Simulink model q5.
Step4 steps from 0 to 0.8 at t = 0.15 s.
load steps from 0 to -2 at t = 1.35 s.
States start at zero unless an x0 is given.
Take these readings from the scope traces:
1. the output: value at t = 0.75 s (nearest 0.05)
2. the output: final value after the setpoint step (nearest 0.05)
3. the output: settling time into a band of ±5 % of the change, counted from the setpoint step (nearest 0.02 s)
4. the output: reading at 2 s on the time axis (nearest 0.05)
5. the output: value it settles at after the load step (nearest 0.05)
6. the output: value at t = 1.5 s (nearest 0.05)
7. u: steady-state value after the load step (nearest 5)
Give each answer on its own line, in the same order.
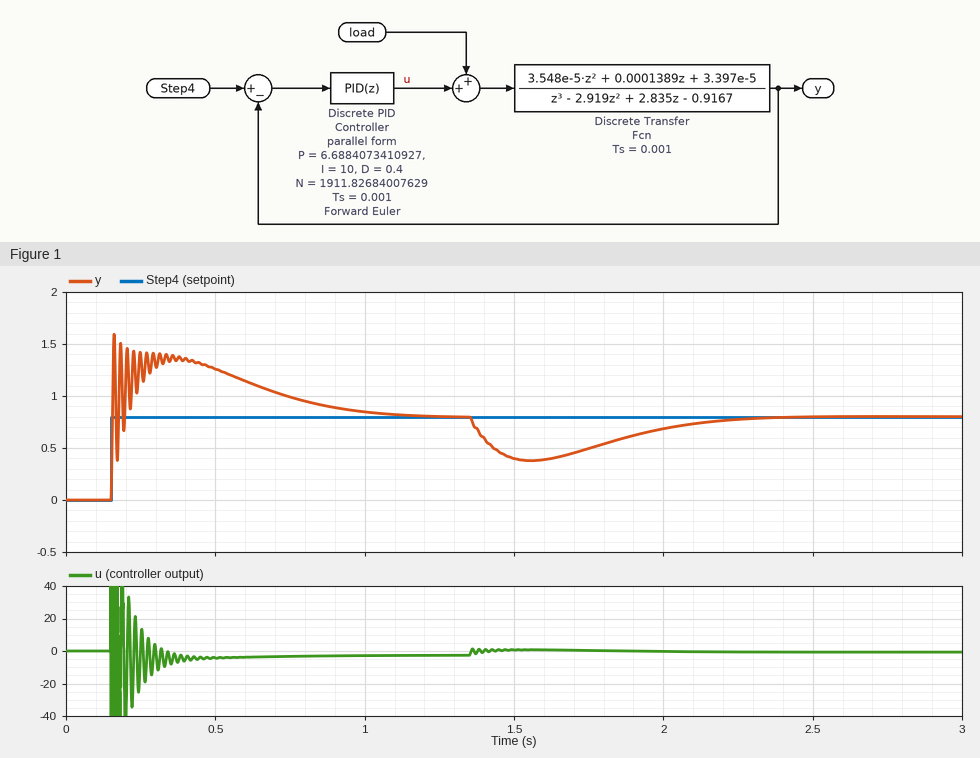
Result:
1.00
0.80
0.88 s
0.70
0.80
0.40
0
